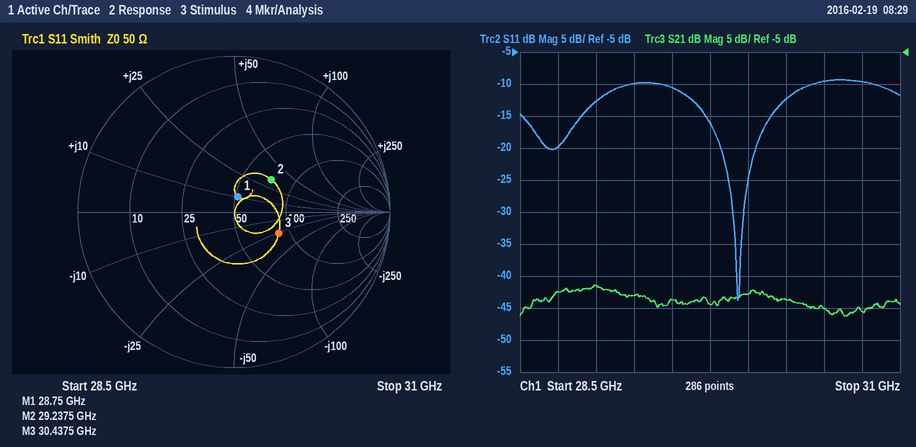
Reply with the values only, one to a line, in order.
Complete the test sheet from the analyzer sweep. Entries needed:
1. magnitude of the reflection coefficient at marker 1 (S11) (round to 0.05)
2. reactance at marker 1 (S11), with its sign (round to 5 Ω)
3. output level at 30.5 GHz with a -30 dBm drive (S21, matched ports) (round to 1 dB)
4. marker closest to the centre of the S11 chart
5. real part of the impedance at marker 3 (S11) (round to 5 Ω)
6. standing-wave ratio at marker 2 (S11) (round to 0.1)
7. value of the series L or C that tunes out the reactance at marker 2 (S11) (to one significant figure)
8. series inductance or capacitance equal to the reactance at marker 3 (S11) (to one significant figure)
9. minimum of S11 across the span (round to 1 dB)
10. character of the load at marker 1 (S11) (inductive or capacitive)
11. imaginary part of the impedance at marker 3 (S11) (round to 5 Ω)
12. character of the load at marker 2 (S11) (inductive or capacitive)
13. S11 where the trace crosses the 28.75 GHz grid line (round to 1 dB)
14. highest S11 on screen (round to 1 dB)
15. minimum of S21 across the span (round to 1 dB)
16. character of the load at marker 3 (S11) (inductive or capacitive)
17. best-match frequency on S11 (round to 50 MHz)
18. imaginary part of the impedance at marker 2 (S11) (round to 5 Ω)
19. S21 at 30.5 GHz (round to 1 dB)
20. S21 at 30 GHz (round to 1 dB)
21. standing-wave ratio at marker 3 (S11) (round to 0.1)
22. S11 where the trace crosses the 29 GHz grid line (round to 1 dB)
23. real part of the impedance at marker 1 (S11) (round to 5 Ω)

0.10
+10 Ω
-75 dBm
marker 1
85 Ω
1.9
200 fF
200 fF
-44 dB
inductive
-25 Ω
inductive
-20 dB
-9 dB
-46 dB
capacitive
29.95 GHz
+35 Ω
-45 dB
-43 dB
1.9
-13 dB
50 Ω
